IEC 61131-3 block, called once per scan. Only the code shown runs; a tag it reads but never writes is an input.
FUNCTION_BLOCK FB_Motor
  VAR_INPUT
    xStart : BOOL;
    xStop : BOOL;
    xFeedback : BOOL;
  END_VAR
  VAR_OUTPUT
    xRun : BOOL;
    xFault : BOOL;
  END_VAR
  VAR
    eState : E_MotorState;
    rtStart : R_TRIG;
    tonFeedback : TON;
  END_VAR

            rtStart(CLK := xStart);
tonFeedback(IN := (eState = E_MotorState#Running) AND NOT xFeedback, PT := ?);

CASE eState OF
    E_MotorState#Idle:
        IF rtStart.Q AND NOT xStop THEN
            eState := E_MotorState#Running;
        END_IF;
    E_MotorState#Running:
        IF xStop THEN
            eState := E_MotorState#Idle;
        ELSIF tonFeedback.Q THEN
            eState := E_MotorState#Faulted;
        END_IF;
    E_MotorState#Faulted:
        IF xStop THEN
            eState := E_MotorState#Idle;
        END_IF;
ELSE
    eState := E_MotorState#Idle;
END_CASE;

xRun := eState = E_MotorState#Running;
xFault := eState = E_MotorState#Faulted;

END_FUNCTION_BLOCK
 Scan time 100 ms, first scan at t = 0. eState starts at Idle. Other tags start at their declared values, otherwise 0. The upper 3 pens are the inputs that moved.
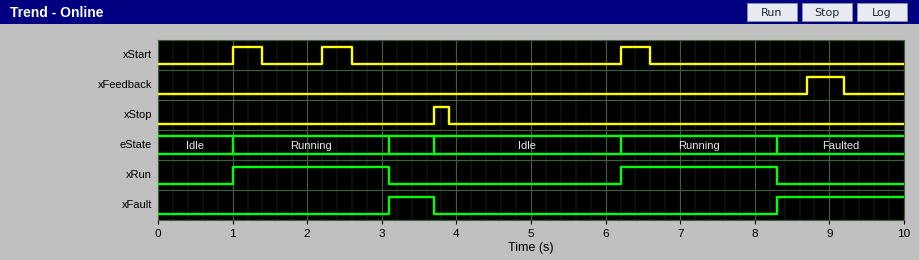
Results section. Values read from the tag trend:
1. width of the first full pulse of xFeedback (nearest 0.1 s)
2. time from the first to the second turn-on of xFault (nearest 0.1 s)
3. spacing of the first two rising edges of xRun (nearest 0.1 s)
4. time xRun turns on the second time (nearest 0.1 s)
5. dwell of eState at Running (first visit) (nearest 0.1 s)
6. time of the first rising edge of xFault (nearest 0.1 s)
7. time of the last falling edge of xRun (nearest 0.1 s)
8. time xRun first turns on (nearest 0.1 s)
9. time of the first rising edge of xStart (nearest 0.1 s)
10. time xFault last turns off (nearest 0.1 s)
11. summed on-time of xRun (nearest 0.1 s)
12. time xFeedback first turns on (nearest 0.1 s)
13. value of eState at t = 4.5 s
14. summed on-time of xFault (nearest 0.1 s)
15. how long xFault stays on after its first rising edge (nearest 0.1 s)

0.5 s
5.2 s
5.2 s
6.2 s
2.1 s
3.1 s
8.3 s
1.0 s
1.0 s
3.7 s
4.2 s
8.7 s
Idle
2.3 s
0.6 s
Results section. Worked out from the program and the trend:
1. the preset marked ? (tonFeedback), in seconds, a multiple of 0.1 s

2.0 s
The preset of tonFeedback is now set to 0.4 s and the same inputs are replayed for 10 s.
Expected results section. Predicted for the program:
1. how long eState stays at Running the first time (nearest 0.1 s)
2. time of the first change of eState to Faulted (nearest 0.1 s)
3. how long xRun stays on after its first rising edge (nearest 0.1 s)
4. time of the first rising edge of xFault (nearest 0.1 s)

0.5 s
1.5 s
0.5 s
1.5 s
